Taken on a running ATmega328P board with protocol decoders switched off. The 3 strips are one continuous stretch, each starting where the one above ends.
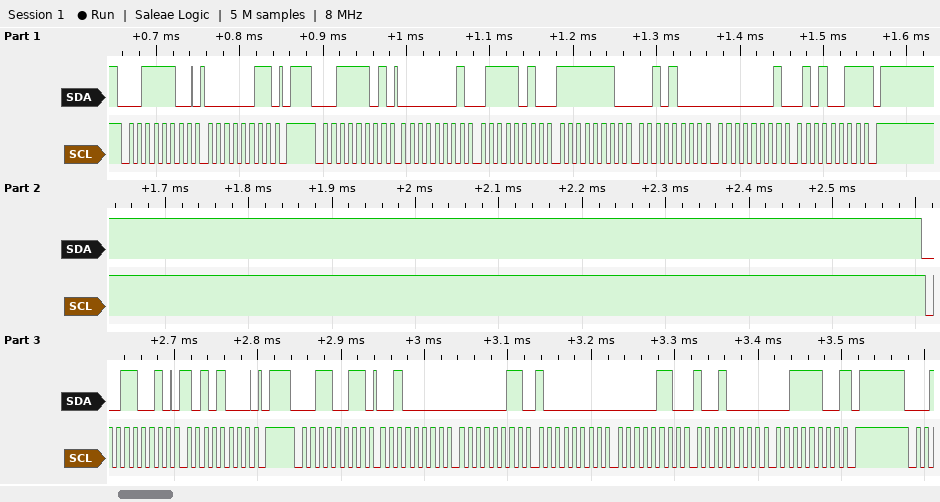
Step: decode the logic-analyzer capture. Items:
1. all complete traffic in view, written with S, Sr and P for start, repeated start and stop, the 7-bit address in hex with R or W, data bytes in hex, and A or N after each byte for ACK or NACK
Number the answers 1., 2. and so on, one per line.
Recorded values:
1. S 1EW A 03 A P S 1ER A 01 A 7A A FE A 28 A 01 A 53 N P S 19W A A8 A P S 19R A 20 A 03 A 80 A 06 A 90 A 3C N P
